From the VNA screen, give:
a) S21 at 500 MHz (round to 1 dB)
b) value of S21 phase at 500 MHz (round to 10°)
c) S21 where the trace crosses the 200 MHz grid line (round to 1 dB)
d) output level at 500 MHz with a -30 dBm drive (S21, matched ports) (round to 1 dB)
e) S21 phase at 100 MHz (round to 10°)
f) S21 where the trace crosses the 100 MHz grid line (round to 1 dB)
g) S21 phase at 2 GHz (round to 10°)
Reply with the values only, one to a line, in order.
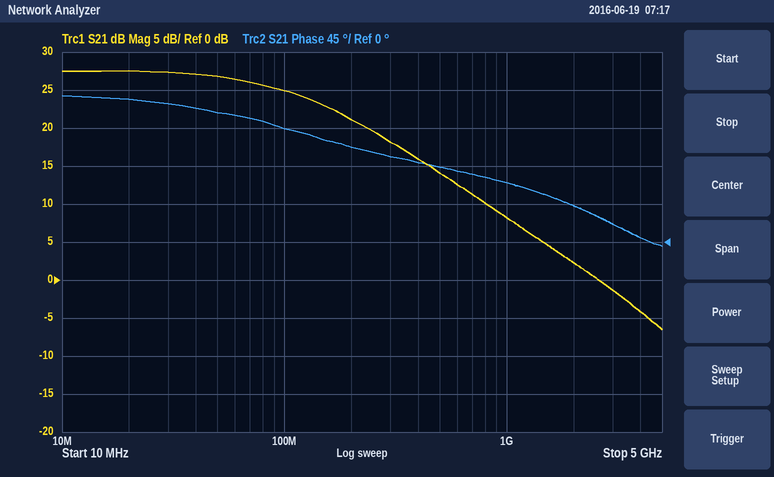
14 dB
90°
21 dB
-16 dBm
130°
25 dB
40°
